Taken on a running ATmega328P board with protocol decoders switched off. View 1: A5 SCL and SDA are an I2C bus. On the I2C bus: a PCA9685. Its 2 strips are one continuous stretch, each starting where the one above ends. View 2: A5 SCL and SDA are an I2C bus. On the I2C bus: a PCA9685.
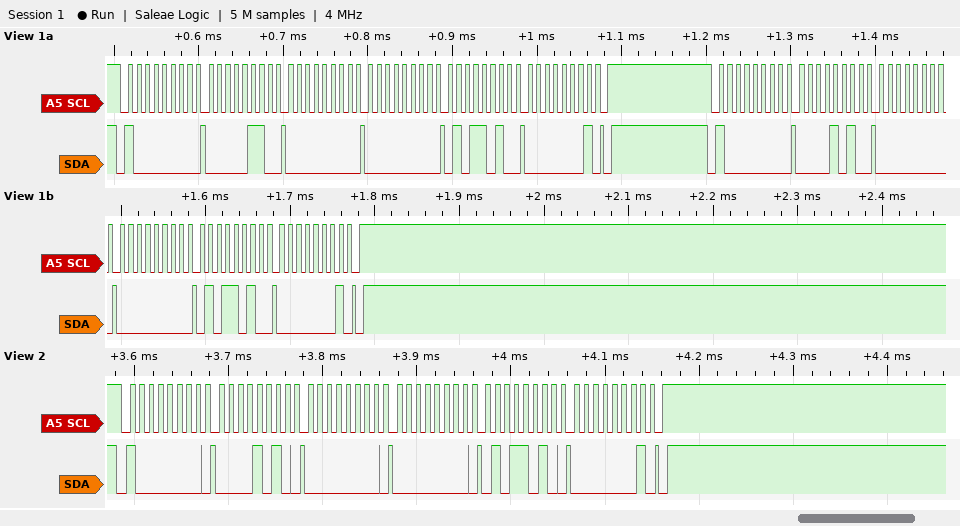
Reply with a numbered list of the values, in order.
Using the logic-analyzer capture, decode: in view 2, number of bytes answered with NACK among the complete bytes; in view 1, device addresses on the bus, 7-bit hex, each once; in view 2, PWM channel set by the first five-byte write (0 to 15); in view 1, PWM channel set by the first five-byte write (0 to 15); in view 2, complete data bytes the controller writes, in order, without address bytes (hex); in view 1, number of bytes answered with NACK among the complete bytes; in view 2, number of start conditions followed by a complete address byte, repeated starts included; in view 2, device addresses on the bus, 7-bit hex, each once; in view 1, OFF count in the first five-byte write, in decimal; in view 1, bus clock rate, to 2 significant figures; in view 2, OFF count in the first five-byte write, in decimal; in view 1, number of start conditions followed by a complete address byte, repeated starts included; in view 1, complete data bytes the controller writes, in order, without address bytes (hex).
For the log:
1. 0
2. 0x40
3. 1
4. 0
5. 0A 00 00 5A 01
6. 0
7. 1
8. 0x40
9. 346
10. 100 kHz
11. 346
12. 2
13. 06 00 00 5A 01 0A 00 00 5A 01
